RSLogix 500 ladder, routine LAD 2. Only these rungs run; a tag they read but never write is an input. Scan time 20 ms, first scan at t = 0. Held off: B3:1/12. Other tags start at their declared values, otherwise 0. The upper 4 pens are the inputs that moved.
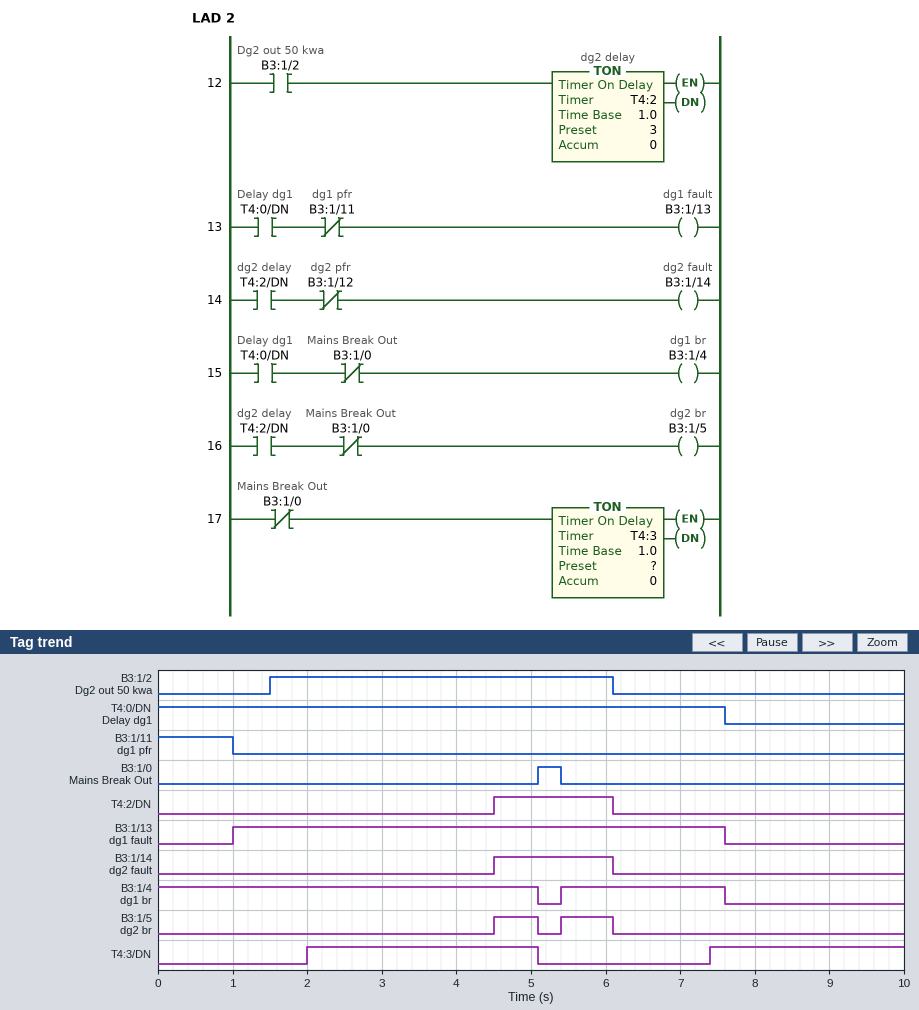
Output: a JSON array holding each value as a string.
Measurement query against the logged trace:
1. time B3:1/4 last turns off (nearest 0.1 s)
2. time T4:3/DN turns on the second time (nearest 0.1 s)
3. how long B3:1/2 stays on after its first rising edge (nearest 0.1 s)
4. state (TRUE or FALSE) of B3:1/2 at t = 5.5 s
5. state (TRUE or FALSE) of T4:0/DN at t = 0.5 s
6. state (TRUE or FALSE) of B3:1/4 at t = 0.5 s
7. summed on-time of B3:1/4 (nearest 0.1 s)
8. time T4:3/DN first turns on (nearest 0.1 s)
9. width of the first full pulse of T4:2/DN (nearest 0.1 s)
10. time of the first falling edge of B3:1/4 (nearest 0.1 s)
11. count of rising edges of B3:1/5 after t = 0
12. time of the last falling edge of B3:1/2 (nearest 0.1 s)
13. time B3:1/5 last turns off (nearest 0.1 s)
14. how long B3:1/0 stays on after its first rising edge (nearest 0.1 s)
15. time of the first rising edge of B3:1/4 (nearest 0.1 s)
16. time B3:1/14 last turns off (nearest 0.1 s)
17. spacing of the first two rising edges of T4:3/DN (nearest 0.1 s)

["7.6 s", "7.4 s", "4.6 s", "TRUE", "TRUE", "TRUE", "7.3 s", "2.0 s", "1.6 s", "5.1 s", "2", "6.1 s", "6.1 s", "0.3 s", "5.4 s", "6.1 s", "5.4 s"]
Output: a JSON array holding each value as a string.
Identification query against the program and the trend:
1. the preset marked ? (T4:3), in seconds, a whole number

["2 s"]
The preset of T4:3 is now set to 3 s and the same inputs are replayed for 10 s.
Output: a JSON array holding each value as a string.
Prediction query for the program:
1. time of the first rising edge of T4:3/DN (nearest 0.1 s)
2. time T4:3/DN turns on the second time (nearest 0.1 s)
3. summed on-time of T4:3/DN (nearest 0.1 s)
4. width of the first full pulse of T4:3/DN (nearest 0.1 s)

["3.0 s", "8.4 s", "3.7 s", "2.1 s"]
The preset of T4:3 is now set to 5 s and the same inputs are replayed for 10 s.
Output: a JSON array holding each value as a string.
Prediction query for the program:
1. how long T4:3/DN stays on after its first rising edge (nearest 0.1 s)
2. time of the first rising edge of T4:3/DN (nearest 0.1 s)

["0.1 s", "5.0 s"]
